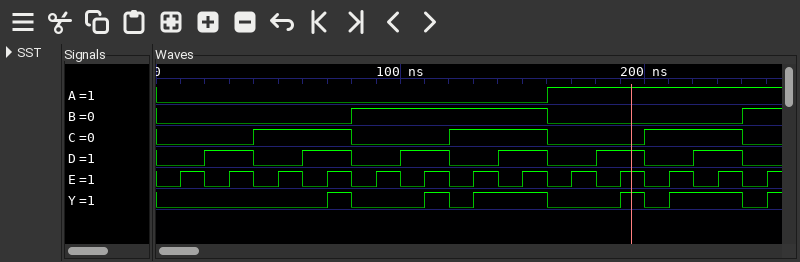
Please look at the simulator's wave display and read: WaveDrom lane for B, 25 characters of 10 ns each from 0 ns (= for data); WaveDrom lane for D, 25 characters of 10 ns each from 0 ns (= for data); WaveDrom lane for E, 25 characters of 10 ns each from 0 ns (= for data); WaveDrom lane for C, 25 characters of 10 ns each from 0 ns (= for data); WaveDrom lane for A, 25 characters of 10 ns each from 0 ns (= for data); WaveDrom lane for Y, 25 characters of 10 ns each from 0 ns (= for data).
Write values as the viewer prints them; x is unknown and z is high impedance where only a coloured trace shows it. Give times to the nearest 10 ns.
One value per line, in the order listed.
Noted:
{name: 'B', wave: '0.......1.......0.......1'}
{name: 'D', wave: '0.1.0.1.0.1.0.1.0.1.0.1.0'}
{name: 'E', wave: '0101010101010101010101010'}
{name: 'C', wave: '0...1...0...1...0...1...0'}
{name: 'A', wave: '0...............1........'}
{name: 'Y', wave: '0......10..101..0..101..0'}
